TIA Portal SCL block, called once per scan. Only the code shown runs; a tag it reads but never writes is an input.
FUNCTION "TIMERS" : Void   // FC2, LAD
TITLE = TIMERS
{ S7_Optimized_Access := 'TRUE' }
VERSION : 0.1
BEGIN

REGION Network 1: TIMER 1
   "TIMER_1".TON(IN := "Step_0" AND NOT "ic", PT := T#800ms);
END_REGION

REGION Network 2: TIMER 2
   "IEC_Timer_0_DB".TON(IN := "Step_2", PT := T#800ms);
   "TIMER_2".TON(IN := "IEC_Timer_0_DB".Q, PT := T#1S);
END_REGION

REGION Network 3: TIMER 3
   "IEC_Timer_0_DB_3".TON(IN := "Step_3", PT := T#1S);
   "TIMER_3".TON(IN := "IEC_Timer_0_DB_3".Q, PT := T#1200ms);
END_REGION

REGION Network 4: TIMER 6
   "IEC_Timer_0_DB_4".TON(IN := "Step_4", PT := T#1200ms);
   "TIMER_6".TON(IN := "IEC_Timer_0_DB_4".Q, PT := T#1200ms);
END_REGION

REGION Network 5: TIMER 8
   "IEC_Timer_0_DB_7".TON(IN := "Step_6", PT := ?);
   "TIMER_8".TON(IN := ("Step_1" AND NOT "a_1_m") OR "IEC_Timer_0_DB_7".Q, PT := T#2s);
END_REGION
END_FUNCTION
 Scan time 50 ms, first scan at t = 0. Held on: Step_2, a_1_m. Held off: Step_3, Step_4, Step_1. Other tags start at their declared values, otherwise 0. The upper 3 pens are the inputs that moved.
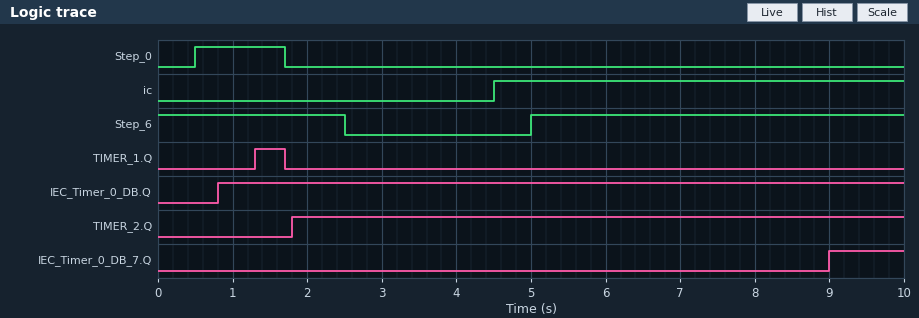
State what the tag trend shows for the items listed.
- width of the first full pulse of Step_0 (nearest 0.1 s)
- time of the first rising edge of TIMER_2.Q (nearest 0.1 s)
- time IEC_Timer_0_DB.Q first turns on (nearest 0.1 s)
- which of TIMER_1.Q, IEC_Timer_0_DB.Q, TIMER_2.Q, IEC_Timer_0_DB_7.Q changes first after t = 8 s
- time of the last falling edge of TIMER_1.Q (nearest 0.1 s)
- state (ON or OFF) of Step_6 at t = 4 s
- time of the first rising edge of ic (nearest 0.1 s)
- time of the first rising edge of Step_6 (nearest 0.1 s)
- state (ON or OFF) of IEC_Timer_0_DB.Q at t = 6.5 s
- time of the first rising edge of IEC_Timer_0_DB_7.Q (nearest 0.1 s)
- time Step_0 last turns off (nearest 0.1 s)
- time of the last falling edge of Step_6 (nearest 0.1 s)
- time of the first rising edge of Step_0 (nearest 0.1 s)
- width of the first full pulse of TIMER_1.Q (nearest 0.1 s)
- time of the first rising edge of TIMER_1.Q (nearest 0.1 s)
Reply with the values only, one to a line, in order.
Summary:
1.2 s
1.8 s
0.8 s
IEC_Timer_0_DB_7.Q
1.7 s
OFF
4.5 s
5.0 s
ON
9.0 s
1.7 s
2.5 s
0.5 s
0.4 s
1.3 s
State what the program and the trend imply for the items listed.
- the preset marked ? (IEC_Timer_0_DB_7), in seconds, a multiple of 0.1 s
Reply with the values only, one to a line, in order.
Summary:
4.0 s
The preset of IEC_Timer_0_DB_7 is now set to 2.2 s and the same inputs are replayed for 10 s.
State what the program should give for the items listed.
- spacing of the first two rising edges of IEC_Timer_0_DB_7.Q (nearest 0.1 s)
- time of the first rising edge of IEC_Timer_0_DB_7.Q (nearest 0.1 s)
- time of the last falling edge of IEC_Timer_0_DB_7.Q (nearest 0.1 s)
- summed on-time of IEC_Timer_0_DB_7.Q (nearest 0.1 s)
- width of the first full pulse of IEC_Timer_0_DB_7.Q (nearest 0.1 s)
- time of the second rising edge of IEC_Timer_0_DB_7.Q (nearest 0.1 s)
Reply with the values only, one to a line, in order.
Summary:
5.0 s
2.2 s
2.5 s
3.1 s
0.3 s
7.2 s
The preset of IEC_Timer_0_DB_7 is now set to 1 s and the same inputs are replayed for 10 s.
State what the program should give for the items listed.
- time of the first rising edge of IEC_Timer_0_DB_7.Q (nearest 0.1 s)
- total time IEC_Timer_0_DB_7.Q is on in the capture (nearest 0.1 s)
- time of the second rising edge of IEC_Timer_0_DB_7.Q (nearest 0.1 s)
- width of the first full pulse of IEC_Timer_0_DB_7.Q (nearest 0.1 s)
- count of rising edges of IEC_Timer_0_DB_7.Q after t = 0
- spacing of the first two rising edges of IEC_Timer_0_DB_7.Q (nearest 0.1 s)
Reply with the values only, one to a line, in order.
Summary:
1.0 s
5.5 s
6.0 s
1.5 s
2
5.0 s
